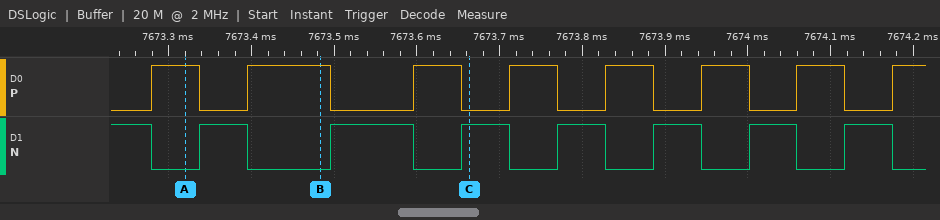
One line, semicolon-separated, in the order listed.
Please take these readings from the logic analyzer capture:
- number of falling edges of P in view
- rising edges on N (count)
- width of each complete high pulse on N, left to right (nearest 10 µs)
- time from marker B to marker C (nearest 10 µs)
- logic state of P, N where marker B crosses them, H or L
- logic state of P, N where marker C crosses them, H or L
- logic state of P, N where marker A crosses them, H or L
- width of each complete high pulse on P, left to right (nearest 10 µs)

7; 7; 60 µs, 100 µs, 60 µs, 60 µs, 60 µs, 60 µs, 60 µs; 180 µs; P=H, N=L; P=L, N=H; P=H, N=L; 60 µs, 100 µs, 60 µs, 60 µs, 60 µs, 60 µs, 60 µs
